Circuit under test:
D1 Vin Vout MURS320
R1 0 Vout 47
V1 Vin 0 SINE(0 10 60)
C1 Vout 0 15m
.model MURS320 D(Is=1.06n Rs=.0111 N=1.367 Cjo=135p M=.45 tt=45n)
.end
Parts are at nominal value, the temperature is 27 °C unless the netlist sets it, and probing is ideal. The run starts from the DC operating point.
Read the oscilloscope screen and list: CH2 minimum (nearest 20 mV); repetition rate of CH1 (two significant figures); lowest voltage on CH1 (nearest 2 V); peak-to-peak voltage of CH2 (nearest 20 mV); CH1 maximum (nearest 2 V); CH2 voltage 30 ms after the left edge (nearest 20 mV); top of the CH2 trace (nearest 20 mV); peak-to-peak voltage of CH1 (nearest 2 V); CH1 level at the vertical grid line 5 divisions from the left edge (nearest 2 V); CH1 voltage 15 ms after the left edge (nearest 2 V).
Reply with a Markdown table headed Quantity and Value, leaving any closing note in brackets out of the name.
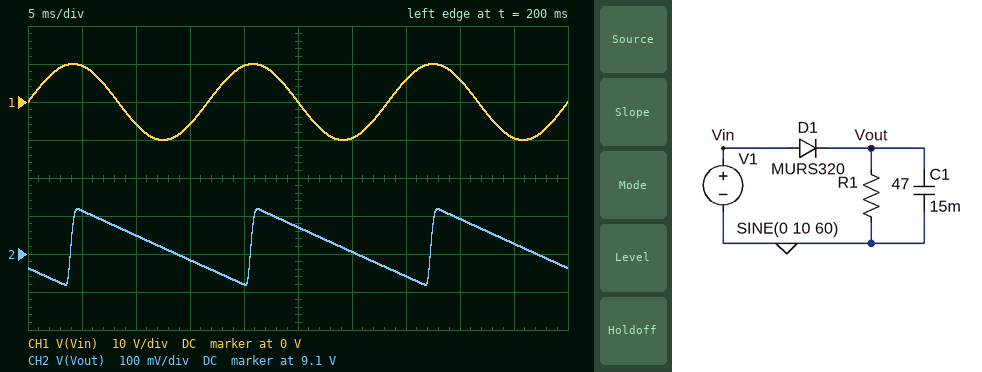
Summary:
| Quantity | Value |
|---|---|
| CH2 minimum | 9.02 V |
| repetition rate of CH1 | 60 Hz |
| lowest voltage on CH1 | -10 V |
| peak-to-peak voltage of CH2 | 200 mV |
| CH1 maximum | 10 V |
| CH2 voltage 30 ms after the left edge | 9.10 V |
| top of the CH2 trace | 9.22 V |
| peak-to-peak voltage of CH1 | 20 V |
| CH1 level at the vertical grid line 5 divisions from the left edge | 0 V |
| CH1 voltage 15 ms after the left edge | -6 V |
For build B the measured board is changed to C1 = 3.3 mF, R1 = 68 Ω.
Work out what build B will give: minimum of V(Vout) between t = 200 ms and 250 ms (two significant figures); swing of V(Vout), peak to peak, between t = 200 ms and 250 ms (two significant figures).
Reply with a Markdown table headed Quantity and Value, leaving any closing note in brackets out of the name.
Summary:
| Quantity | Value |
|---|---|
| minimum of V(Vout) between t = 200 ms and 250 ms | 8.7 V |
| swing of V(Vout), peak to peak, between t = 200 ms and 250 ms | 610 mV |
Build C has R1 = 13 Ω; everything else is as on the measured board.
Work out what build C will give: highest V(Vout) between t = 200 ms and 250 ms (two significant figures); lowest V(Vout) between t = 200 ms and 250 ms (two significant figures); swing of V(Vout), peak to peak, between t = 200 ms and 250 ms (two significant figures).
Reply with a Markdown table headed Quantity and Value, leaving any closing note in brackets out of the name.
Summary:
| Quantity | Value |
|---|---|
| highest V(Vout) between t = 200 ms and 250 ms | 9.2 V |
| lowest V(Vout) between t = 200 ms and 250 ms | 8.5 V |
| swing of V(Vout), peak to peak, between t = 200 ms and 250 ms | 690 mV |
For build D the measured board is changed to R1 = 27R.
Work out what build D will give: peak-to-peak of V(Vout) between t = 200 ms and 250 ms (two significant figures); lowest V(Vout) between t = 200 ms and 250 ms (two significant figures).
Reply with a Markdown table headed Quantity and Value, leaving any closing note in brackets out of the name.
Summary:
| Quantity | Value |
|---|---|
| peak-to-peak of V(Vout) between t = 200 ms and 250 ms | 340 mV |
| lowest V(Vout) between t = 200 ms and 250 ms | 8.9 V |
